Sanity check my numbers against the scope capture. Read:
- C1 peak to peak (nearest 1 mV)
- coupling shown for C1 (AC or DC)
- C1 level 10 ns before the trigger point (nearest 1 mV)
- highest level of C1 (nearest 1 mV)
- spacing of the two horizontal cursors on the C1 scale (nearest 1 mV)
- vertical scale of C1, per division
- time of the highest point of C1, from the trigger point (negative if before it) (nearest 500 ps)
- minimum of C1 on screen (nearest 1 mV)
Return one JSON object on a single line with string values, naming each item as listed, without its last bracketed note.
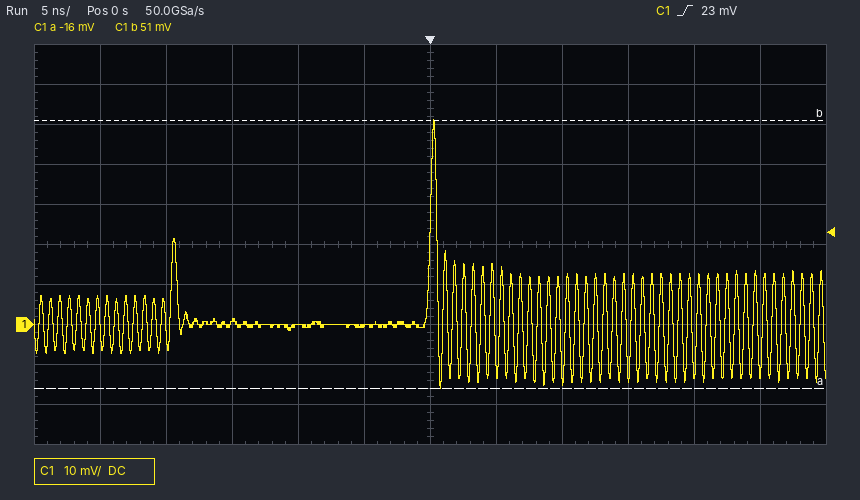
{"C1 peak to peak": "67 mV", "coupling shown for C1": "DC", "C1 level 10 ns before the trigger point": "0 mV", "highest level of C1": "51 mV", "spacing of the two horizontal cursors on the C1 scale": "67 mV", "vertical scale of C1, per division": "10 mV", "time of the highest point of C1, from the trigger point (negative if before it)": "+500 ps", "minimum of C1 on screen": "-16 mV"}
